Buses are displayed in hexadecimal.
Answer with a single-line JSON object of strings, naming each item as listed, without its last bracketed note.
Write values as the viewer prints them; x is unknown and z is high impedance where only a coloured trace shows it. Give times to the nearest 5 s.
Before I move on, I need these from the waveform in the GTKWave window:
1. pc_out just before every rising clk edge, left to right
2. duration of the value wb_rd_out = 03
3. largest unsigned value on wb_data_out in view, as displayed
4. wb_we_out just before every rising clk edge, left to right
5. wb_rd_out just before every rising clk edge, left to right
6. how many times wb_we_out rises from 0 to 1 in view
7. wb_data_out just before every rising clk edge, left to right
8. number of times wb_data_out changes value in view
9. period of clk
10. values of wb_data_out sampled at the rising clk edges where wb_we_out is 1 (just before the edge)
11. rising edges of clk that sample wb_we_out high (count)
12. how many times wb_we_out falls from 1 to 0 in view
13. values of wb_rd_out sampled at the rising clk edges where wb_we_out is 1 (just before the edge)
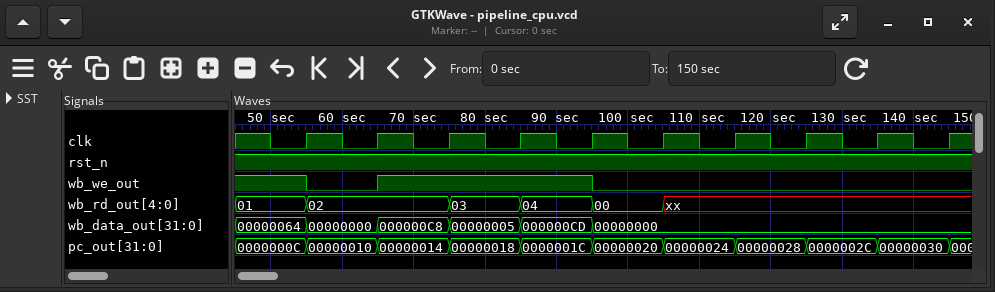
{"pc_out just before every rising clk edge, left to right": "0000000C, 00000010, 00000014, 00000018, 0000001C, 00000020, 00000024, 00000028, 0000002C, 00000030", "duration of the value wb_rd_out = 03": "10 s", "largest unsigned value on wb_data_out in view, as displayed": "000000CD", "wb_we_out just before every rising clk edge, left to right": "1 0 1 1 1 0 0 0 0 0", "wb_rd_out just before every rising clk edge, left to right": "01, 02, 02, 03, 04, 00, xx, xx, xx, xx", "how many times wb_we_out rises from 0 to 1 in view": "1", "wb_data_out just before every rising clk edge, left to right": "00000064, 00000000, 000000C8, 00000005, 000000CD, 00000000, 00000000, 00000000, 00000000, 00000000", "number of times wb_data_out changes value in view": "5", "period of clk": "10 s", "values of wb_data_out sampled at the rising clk edges where wb_we_out is 1": "00000064, 000000C8, 00000005, 000000CD", "rising edges of clk that sample wb_we_out high": "4", "how many times wb_we_out falls from 1 to 0 in view": "2", "values of wb_rd_out sampled at the rising clk edges where wb_we_out is 1": "01, 02, 03, 04"}
